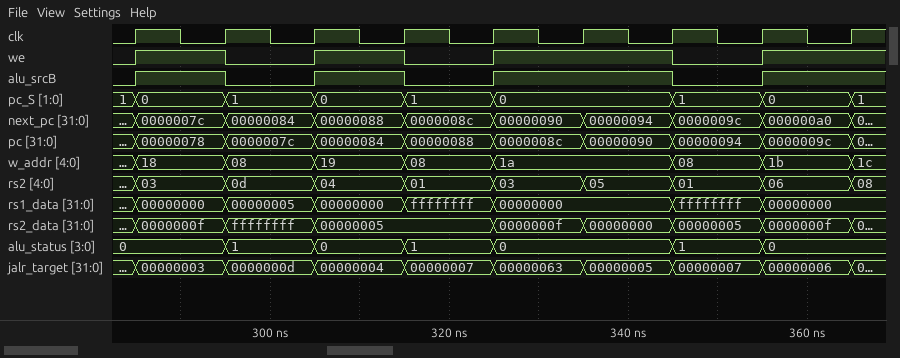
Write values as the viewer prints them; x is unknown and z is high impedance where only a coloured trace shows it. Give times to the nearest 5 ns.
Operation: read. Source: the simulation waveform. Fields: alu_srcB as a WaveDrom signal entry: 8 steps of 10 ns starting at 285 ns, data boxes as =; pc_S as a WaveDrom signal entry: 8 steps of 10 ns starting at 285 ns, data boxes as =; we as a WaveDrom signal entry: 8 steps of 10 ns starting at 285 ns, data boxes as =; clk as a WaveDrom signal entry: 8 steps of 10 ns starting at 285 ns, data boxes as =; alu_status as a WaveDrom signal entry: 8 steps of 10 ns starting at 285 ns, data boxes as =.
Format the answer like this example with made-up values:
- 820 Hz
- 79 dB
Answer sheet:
- {name: 'alu_srcB', wave: '10101.01'}
- {name: 'pc_S', wave: '=====.==', data: '0 1 0 1 0 1 0'}
- {name: 'we', wave: '10101.01'}
- {name: 'clk', wave: 'p.......'}
- {name: 'alu_status', wave: '=====.==', data: '0 1 0 1 0 1 0'}
